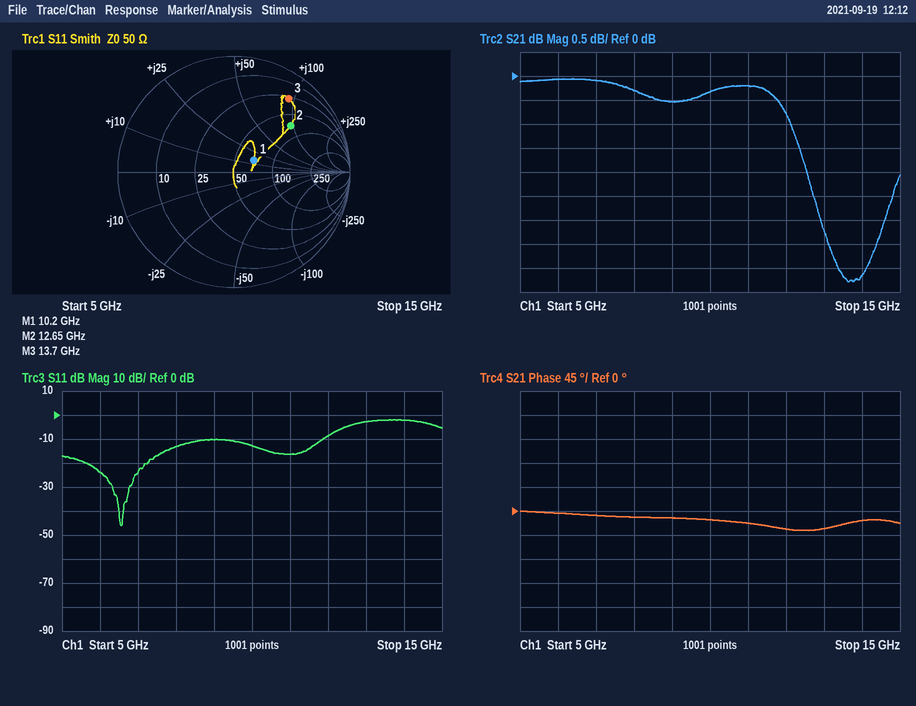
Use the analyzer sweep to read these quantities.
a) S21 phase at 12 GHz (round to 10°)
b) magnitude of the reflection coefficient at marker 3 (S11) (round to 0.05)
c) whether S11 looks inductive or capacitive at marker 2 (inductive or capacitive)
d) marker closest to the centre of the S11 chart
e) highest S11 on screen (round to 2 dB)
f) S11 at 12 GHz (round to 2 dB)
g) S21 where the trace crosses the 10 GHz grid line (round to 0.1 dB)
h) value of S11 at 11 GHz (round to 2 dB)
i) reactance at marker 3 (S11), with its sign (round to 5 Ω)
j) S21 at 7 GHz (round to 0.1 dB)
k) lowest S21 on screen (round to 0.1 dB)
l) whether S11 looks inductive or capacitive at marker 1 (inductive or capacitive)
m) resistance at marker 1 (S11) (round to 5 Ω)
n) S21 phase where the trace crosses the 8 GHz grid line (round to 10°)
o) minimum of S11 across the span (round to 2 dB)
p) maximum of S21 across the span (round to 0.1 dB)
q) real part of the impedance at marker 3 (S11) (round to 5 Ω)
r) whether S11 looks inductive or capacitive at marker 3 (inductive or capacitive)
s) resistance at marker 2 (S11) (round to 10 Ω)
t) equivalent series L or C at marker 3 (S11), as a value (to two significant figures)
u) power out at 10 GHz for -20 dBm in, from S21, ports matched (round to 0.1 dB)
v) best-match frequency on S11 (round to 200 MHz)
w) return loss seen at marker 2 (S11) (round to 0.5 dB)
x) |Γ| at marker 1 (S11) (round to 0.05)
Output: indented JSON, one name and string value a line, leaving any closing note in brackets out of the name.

{
  "S21 phase at 12 GHz": "-30°",
  "magnitude of the reflection coefficient at marker 3 (S11)": "0.80",
  "whether S11 looks inductive or capacitive at marker 2": "inductive",
  "marker closest to the centre of the S11 chart": "marker 1",
  "highest S11 on screen": "-2 dB",
  "S11 at 12 GHz": "-8 dB",
  "S21 where the trace crosses the 10 GHz grid line": "-0.3 dB",
  "value of S11 at 11 GHz": "-16 dB",
  "reactance at marker 3 (S11), with its sign": "+95 Ω",
  "S21 at 7 GHz": "-0.1 dB",
  "lowest S21 on screen": "-4.3 dB",
  "whether S11 looks inductive or capacitive at marker 1": "inductive",
  "resistance at marker 1 (S11)": "70 Ω",
  "S21 phase where the trace crosses the 8 GHz grid line": "-10°",
  "minimum of S11 across the span": "-46 dB",
  "maximum of S21 across the span": "-0.1 dB",
  "real part of the impedance at marker 3 (S11)": "30 Ω",
  "whether S11 looks inductive or capacitive at marker 3": "inductive",
  "resistance at marker 2 (S11)": "70 Ω",
  "equivalent series L or C at marker 3 (S11), as a value": "1.1 nH",
  "power out at 10 GHz for -20 dBm in, from S21, ports matched": "-20.3 dBm",
  "best-match frequency on S11": "6.6 GHz",
  "return loss seen at marker 2 (S11)": "4.0 dB",
  "|Γ| at marker 1 (S11)": "0.20"
}
